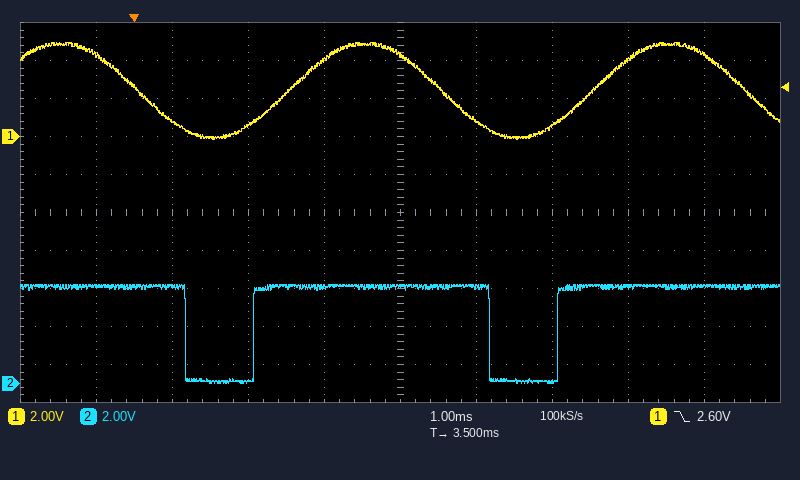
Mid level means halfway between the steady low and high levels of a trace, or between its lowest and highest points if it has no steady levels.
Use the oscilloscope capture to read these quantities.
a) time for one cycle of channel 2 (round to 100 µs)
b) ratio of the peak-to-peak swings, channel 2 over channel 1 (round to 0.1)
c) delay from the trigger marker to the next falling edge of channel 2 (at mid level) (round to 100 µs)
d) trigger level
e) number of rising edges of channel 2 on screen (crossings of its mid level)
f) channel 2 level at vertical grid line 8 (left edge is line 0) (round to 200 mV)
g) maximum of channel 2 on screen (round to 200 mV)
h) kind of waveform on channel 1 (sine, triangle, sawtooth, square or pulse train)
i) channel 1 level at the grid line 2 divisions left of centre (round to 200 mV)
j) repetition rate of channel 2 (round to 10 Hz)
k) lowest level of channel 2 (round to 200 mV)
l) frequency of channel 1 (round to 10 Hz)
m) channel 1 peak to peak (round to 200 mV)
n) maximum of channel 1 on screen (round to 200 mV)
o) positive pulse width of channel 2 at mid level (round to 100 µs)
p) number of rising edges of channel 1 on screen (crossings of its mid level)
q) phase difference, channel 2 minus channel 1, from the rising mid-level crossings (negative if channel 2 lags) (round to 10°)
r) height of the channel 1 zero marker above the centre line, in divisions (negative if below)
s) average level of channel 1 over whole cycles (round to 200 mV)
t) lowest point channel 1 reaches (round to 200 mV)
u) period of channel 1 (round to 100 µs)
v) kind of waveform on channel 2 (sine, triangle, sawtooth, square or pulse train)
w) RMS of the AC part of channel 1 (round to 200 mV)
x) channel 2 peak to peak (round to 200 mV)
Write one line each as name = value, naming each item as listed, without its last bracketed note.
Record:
time for one cycle of channel 2 = 4.0 ms
ratio of the peak-to-peak swings, channel 2 over channel 1 = 1.0
delay from the trigger marker to the next falling edge of channel 2 (at mid level) = 700 µs
trigger level = 2.60 V
number of rising edges of channel 2 on screen = 2
channel 2 level at vertical grid line 8 (left edge is line 0) = 5.0 V
maximum of channel 2 on screen = 5.2 V
kind of waveform on channel 1 = sine
channel 1 level at the grid line 2 divisions left of centre = 600 mV
repetition rate of channel 2 = 250 Hz
lowest level of channel 2 = 0.0 V
frequency of channel 1 = 250 Hz
channel 1 peak to peak = 5.2 V
maximum of channel 1 on screen = 5.0 V
positive pulse width of channel 2 at mid level = 3.1 ms
number of rising edges of channel 1 on screen = 2
phase difference, channel 2 minus channel 1, from the rising mid-level crossings (negative if channel 2 lags) = +40°
height of the channel 1 zero marker above the centre line, in divisions = +2.0 div
average level of channel 1 over whole cycles = 2.4 V
lowest point channel 1 reaches = -200 mV
period of channel 1 = 4.0 ms
kind of waveform on channel 2 = pulse train
RMS of the AC part of channel 1 = 1.8 V
channel 2 peak to peak = 5.2 V
